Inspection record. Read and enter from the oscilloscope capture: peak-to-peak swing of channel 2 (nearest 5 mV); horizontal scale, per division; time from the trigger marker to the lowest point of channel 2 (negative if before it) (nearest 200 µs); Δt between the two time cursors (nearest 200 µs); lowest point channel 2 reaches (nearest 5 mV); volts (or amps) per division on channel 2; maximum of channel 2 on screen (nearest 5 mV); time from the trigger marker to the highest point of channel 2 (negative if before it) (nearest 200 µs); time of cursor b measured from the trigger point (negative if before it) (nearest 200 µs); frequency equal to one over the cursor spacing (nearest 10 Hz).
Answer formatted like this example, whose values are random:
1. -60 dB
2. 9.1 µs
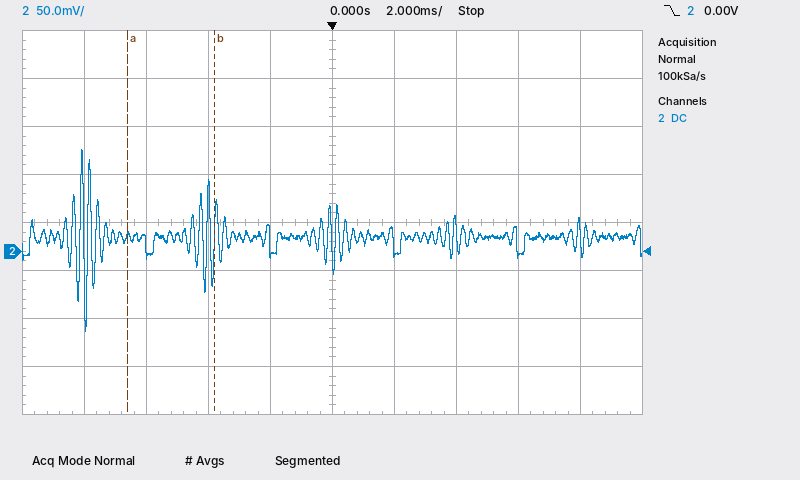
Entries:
1. 190 mV
2. 2 ms
3. -8.0 ms
4. 2.8 ms
5. -85 mV
6. 50 mV
7. 105 mV
8. -8.0 ms
9. -3.8 ms
10. 360 Hz
